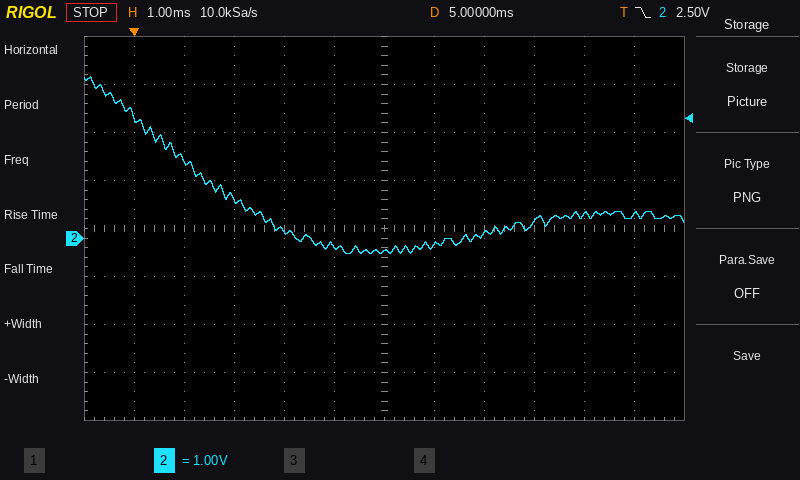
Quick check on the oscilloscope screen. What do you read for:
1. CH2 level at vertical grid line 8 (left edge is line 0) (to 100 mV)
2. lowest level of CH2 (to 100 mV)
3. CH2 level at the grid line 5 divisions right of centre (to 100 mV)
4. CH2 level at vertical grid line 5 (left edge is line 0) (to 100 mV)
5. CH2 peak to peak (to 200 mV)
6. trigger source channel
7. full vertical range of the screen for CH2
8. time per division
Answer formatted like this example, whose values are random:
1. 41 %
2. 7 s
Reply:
1. 100 mV
2. -300 mV
3. 500 mV
4. -200 mV
5. 3.6 V
6. CH2
7. 8 V
8. 1 ms
